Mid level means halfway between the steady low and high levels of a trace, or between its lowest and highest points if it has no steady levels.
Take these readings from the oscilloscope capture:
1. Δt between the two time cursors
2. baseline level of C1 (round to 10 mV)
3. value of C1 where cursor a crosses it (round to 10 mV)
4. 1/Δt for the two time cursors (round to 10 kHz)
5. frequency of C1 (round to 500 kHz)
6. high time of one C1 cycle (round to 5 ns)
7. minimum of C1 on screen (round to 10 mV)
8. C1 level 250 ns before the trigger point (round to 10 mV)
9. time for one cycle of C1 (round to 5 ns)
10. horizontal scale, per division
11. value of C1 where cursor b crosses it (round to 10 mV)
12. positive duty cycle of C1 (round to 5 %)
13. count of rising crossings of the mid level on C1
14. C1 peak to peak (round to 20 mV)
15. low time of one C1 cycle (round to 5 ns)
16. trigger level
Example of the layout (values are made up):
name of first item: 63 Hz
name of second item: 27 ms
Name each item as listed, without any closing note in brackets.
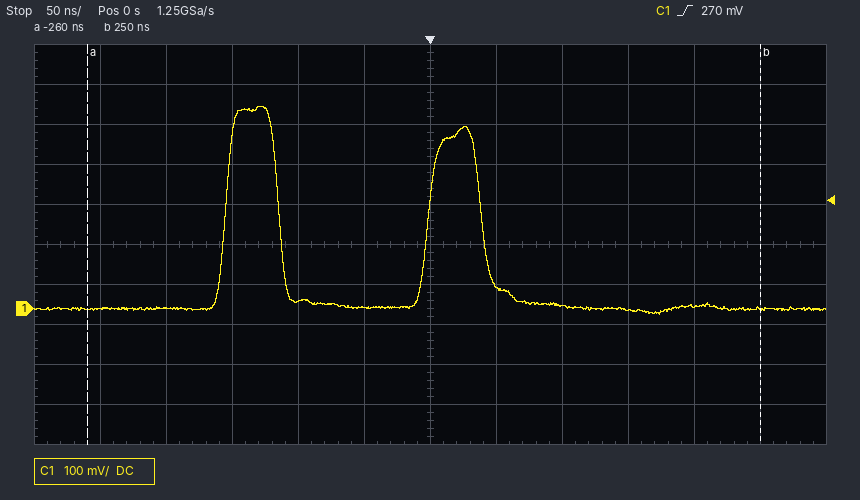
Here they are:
Δt between the two time cursors: 510 ns
baseline level of C1: 0 mV
value of C1 where cursor a crosses it: 0 mV
1/Δt for the two time cursors: 1.96 MHz
frequency of C1: 6.5 MHz
high time of one C1 cycle: 40 ns
minimum of C1 on screen: -10 mV
C1 level 250 ns before the trigger point: 0 mV
time for one cycle of C1: 155 ns
horizontal scale, per division: 50 ns
value of C1 where cursor b crosses it: 0 mV
positive duty cycle of C1: 25 %
count of rising crossings of the mid level on C1: 2
C1 peak to peak: 520 mV
low time of one C1 cycle: 115 ns
trigger level: 270 mV
